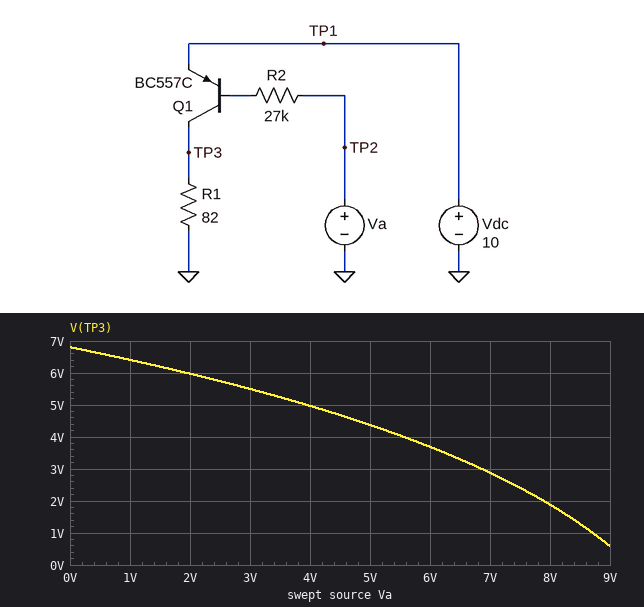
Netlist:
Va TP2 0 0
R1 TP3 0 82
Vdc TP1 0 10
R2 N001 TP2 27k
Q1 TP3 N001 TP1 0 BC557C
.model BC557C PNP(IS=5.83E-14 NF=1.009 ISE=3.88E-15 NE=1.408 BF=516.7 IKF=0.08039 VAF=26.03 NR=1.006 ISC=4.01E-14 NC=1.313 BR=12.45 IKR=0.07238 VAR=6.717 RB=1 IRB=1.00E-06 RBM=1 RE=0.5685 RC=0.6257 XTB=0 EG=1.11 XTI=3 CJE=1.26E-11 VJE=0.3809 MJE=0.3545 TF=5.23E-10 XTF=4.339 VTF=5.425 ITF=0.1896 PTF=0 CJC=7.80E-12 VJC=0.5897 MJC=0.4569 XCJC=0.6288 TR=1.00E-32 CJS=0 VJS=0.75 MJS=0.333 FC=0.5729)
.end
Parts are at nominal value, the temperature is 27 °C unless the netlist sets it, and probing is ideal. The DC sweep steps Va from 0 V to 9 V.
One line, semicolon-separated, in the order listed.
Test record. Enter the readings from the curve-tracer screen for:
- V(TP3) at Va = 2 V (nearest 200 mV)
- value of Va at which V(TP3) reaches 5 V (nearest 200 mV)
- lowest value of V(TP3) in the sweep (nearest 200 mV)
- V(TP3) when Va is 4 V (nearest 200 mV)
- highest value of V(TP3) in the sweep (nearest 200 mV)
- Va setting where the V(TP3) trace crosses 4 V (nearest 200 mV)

6.0 V; 4.0 V; 600 mV; 5.0 V; 6.8 V; 5.6 V
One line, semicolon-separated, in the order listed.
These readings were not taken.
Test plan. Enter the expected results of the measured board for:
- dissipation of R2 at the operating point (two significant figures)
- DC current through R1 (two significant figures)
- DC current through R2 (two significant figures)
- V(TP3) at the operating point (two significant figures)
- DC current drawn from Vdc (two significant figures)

3.1 mW; 83 mA; 340 µA; 6.8 V; 83 mA
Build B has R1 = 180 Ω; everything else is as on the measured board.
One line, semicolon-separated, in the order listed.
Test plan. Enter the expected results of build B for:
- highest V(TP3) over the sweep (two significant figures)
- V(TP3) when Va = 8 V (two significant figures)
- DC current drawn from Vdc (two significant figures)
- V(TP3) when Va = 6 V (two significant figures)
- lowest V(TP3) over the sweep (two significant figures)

9.8 V; 3.9 V; 55 mA; 7.1 V; 1.3 V
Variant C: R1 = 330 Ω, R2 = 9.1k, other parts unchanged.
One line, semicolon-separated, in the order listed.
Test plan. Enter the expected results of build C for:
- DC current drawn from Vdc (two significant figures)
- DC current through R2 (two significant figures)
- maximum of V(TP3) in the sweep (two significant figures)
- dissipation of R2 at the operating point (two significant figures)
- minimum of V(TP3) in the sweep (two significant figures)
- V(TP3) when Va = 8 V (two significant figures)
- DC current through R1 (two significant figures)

31 mA; 1.0 mA; 9.9 V; 9.4 mW; 5.0 V; 9.8 V; 30 mA
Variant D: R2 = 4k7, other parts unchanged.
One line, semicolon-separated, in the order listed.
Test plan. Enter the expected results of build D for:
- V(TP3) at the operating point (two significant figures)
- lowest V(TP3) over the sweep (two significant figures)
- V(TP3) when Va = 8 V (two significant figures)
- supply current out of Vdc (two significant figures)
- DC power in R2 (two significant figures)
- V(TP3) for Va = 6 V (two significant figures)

9.8 V; 2.2 V; 5.9 V; 120 mA; 18 mW; 9.4 V
